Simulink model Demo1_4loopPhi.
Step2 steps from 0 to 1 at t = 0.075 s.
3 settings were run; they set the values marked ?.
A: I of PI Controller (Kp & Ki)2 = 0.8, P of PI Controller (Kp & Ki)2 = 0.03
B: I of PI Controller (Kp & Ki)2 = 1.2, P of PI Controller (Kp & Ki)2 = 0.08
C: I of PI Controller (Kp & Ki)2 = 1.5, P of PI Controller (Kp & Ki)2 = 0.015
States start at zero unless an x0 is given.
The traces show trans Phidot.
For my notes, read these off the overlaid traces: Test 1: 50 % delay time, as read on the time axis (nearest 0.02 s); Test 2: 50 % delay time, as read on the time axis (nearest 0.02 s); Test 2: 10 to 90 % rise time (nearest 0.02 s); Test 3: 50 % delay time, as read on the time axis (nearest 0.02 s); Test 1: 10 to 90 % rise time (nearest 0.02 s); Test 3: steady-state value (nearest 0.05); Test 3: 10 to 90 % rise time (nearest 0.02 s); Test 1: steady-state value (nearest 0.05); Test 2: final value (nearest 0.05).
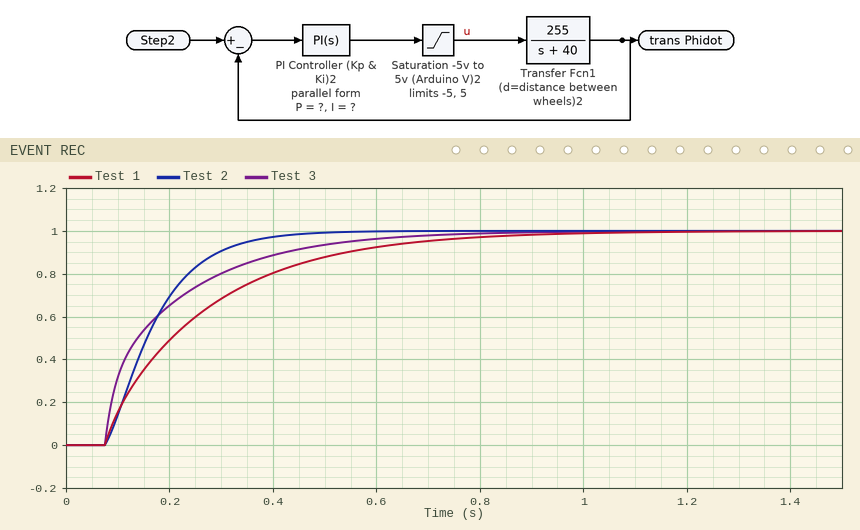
0.20 s
0.16 s
0.20 s
0.14 s
0.46 s
1.00
0.34 s
1.00
1.00
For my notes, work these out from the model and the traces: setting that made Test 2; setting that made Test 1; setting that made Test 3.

C
A
B
